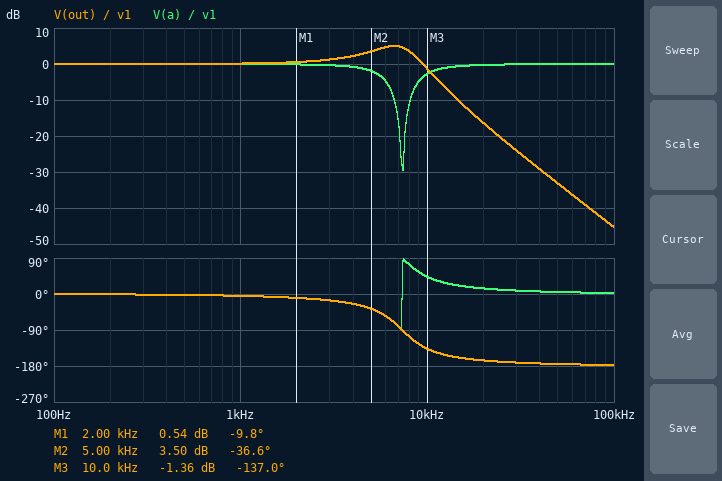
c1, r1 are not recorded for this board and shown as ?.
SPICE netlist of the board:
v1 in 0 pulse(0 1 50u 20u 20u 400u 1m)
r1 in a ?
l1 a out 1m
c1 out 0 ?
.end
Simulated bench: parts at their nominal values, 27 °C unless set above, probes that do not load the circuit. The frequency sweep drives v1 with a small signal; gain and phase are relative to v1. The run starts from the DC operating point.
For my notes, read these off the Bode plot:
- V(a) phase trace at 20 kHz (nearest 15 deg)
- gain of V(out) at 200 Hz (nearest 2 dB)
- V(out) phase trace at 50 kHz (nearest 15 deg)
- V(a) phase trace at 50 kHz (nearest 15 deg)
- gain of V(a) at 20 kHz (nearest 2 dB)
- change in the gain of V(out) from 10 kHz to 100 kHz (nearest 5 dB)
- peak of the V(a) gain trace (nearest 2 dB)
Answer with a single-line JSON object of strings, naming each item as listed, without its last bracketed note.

{"V(a) phase trace at 20 kHz": "15 deg", "gain of V(out) at 200 Hz": "0 dB", "V(out) phase trace at 50 kHz": "-180 deg", "V(a) phase trace at 50 kHz": "0 deg", "gain of V(a) at 20 kHz": "0 dB", "change in the gain of V(out) from 10 kHz to 100 kHz": "-45 dB", "peak of the V(a) gain trace": "0 dB"}
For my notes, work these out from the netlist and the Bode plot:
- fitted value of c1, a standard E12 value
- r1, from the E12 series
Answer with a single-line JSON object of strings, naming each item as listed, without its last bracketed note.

{"fitted value of c1, a standard E12 value": "470 nF", "r1, from the E12 series": "27 Ω"}
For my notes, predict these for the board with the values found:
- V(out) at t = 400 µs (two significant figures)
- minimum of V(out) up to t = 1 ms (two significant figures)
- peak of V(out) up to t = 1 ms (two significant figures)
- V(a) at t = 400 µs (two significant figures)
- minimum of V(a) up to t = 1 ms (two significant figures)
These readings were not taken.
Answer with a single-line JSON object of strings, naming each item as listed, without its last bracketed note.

{"V(out) at t = 400 µs": "1.0 V", "minimum of V(out) up to t = 1 ms": "-370 mV", "peak of V(out) up to t = 1 ms": "1.4 V", "V(a) at t = 400 µs": "1.0 V", "minimum of V(a) up to t = 1 ms": "-150 mV"}
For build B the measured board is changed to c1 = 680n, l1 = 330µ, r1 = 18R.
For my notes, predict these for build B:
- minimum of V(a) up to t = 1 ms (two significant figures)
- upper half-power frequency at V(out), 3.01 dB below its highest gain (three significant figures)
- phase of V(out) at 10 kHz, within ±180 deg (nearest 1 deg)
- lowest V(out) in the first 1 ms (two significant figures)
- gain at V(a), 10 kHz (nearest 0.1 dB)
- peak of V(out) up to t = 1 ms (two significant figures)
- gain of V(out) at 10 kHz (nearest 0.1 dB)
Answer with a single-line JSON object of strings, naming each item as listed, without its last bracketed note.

{"minimum of V(a) up to t = 1 ms": "-110 mV", "upper half-power frequency at V(out), 3.01 dB below its highest gain": "12.6 kHz", "phase of V(out) at 10 kHz, within ±180 deg": "-82 deg", "lowest V(out) in the first 1 ms": "-230 mV", "gain at V(a), 10 kHz": "-16.7 dB", "peak of V(out) up to t = 1 ms": "1.2 V", "gain of V(out) at 10 kHz": "2.2 dB"}
